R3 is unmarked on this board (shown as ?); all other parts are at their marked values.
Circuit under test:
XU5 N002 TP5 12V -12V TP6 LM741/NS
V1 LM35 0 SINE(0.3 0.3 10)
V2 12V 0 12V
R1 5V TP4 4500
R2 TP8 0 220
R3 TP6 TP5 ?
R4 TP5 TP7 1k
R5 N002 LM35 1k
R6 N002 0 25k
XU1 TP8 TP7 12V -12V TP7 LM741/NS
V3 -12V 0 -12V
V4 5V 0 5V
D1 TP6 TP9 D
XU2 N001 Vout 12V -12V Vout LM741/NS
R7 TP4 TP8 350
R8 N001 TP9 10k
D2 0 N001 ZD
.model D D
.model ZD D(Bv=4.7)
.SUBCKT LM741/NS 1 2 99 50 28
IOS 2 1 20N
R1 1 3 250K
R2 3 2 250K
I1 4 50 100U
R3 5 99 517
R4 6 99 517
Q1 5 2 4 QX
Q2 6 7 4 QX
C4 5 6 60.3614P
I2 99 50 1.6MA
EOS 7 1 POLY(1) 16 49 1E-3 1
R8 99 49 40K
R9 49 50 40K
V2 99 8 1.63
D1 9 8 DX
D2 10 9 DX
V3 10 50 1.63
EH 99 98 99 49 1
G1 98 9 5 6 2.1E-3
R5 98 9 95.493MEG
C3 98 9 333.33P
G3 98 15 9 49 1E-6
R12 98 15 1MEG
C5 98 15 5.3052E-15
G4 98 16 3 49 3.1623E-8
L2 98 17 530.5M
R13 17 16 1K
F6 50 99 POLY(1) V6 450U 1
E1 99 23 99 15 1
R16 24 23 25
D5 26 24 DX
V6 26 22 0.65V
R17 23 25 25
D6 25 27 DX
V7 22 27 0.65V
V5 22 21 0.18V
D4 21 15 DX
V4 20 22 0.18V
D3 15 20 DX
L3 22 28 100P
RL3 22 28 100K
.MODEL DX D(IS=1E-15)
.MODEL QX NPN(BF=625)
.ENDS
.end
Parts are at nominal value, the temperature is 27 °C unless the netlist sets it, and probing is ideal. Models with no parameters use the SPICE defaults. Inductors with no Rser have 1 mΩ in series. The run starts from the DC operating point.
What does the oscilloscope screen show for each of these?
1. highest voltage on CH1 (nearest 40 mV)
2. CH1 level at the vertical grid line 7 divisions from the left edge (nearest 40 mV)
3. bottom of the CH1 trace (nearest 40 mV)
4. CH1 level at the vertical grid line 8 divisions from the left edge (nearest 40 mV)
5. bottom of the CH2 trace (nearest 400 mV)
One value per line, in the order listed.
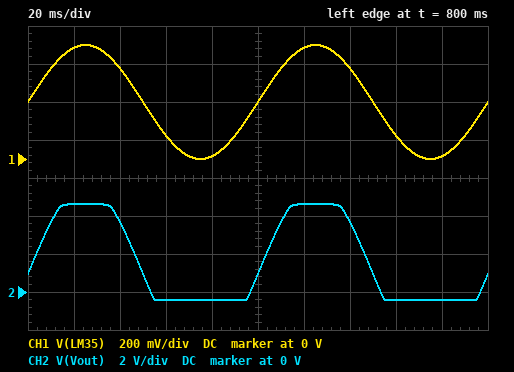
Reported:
600 mV
480 mV
0 V
120 mV
-400 mV
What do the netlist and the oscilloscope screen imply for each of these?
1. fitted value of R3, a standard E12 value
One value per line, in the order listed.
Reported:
15 kΩ
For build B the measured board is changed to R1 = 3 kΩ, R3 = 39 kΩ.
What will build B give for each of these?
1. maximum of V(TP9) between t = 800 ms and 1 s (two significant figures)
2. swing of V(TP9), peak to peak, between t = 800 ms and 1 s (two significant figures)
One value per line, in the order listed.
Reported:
10 V
11 V
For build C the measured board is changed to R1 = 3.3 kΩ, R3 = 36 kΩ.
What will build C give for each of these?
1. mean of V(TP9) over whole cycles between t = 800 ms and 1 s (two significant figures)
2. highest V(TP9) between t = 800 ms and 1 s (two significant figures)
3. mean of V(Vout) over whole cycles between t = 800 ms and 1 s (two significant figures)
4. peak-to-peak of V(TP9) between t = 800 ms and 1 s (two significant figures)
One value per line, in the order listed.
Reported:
3.1 V
10 V
1.8 V
11 V
